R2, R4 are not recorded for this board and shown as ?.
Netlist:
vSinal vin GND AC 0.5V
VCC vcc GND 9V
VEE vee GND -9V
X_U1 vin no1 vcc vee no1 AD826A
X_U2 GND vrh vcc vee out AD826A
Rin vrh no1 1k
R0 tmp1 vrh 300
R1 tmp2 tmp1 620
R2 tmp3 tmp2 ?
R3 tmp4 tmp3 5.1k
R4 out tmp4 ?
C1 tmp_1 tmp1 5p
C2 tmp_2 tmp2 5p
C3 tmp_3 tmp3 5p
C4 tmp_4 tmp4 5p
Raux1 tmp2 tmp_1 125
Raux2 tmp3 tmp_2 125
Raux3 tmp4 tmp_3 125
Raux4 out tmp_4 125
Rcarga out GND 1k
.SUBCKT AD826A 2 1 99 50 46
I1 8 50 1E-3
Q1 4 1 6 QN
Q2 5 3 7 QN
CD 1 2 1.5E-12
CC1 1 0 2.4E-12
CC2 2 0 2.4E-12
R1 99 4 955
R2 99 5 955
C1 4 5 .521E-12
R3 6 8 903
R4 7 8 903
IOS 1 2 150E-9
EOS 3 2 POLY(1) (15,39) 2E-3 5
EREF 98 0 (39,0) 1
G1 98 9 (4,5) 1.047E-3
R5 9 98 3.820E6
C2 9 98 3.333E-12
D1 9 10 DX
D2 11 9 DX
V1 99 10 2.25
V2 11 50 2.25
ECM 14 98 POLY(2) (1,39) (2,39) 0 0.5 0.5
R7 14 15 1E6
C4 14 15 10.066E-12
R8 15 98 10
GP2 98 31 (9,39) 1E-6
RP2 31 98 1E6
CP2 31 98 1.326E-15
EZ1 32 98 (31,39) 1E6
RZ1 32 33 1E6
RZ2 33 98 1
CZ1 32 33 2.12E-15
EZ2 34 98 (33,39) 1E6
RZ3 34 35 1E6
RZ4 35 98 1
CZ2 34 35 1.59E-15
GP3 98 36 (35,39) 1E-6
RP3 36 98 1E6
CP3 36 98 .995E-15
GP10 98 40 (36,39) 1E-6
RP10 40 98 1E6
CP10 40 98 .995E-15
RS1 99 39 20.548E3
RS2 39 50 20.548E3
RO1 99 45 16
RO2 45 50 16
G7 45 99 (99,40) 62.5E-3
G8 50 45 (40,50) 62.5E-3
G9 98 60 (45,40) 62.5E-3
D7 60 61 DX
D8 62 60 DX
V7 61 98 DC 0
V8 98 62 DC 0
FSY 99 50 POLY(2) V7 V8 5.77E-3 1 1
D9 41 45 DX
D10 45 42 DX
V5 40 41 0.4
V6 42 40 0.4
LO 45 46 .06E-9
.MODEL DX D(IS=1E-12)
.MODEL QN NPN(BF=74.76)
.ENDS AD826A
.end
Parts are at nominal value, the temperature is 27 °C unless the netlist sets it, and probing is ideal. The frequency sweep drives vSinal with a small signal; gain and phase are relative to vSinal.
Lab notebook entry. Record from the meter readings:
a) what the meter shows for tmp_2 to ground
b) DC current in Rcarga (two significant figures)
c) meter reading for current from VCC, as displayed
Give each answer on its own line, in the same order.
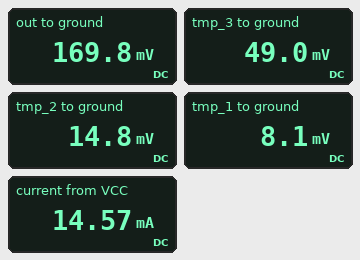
14.8 mV
170 µA
14.57 mA
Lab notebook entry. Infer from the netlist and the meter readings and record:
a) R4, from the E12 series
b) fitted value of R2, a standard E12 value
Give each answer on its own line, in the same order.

18 kΩ
1 kΩ
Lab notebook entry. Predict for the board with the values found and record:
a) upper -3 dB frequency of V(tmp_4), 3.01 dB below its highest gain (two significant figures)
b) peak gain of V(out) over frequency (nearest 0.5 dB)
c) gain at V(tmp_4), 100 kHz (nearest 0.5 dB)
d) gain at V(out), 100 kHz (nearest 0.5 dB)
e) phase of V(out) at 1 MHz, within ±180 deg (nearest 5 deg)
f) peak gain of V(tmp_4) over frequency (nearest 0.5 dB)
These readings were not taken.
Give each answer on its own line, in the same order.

1.0 MHz
28.0 dB
28.0 dB
28.0 dB
135 deg
28.0 dB
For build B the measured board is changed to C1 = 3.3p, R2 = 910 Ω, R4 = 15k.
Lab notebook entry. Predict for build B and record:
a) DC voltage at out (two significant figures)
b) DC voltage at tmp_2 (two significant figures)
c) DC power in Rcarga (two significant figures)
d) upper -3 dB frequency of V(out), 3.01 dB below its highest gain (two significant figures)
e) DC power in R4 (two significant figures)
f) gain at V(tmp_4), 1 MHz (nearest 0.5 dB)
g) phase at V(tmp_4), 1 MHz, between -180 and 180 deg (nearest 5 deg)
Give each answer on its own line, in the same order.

150 mV
14 mV
22 µW
1.2 MHz
680 nW
24.5 dB
140 deg
